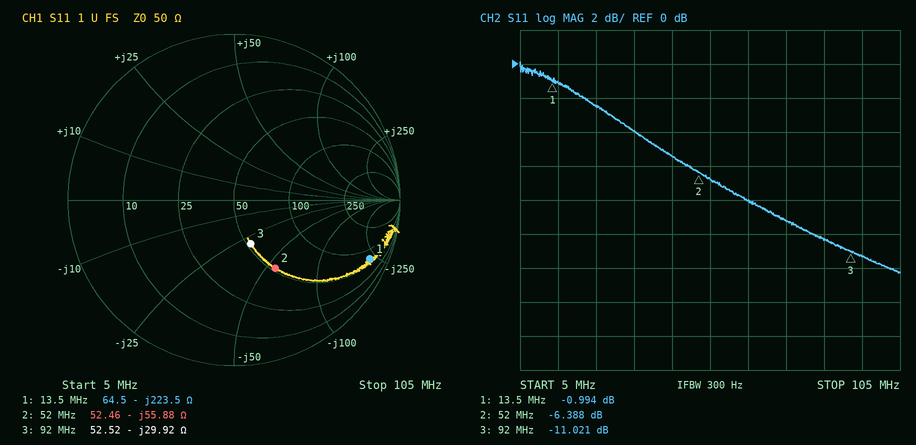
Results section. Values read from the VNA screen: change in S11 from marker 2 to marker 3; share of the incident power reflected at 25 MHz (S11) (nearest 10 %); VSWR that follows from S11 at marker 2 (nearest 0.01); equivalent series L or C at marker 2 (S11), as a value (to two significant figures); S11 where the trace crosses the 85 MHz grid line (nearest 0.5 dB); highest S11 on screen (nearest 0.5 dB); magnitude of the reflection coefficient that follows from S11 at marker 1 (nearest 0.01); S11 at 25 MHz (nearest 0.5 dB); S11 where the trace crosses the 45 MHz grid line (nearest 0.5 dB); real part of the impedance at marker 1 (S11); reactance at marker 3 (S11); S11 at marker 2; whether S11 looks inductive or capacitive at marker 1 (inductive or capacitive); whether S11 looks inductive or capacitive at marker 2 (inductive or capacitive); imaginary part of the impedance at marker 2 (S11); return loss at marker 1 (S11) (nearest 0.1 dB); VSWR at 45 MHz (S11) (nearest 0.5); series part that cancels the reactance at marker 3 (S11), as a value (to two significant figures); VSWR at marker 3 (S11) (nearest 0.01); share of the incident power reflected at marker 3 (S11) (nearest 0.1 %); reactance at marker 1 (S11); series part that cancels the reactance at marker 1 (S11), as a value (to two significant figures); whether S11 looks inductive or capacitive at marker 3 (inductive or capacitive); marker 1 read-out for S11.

-4.633 dB
60 %
2.84
55 pF
-10.5 dB
0.0 dB
0.89
-2.5 dB
-5.5 dB
64.5 Ω
-29.92 Ω
-6.388 dB
capacitive
capacitive
-55.88 Ω
1.0 dB
3.5
52 nH
1.78
7.9 %
-223.5 Ω
2.6 µH
capacitive
-0.994 dB
